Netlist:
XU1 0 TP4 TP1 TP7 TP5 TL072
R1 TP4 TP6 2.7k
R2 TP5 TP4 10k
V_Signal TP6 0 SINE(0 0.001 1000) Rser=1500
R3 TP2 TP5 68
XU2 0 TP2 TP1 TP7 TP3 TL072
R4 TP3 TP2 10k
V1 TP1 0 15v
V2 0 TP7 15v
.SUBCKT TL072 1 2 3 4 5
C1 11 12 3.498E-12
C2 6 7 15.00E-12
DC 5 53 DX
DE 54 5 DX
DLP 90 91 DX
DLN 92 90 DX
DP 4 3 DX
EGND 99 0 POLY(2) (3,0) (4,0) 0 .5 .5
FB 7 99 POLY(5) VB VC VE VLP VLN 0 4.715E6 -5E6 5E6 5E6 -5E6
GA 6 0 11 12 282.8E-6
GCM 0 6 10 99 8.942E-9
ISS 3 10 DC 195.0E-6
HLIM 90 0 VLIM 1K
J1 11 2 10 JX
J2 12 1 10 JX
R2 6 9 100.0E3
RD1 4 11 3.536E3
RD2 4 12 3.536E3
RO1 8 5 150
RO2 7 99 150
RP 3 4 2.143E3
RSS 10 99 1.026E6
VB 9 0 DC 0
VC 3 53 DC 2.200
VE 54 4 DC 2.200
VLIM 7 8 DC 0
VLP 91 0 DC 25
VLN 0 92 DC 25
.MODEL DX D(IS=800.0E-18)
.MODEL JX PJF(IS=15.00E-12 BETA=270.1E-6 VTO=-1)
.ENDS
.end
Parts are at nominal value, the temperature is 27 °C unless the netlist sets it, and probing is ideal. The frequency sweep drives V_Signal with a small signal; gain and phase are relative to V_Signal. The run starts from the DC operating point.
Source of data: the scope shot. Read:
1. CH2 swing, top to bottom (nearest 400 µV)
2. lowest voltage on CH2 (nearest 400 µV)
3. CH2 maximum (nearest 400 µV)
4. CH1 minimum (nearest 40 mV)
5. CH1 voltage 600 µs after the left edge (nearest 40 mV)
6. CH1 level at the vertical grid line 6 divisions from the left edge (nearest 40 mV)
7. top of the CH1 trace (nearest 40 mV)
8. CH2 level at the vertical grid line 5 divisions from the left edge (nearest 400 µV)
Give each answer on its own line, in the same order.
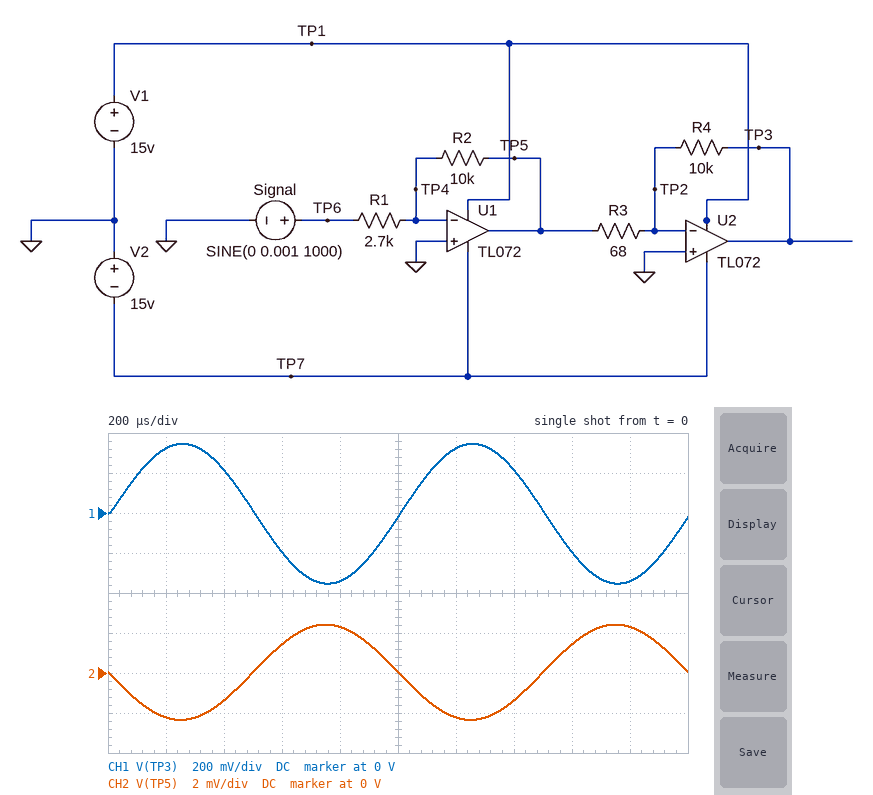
4.8 mV
-2.4 mV
2.4 mV
-360 mV
-200 mV
320 mV
360 mV
0 V
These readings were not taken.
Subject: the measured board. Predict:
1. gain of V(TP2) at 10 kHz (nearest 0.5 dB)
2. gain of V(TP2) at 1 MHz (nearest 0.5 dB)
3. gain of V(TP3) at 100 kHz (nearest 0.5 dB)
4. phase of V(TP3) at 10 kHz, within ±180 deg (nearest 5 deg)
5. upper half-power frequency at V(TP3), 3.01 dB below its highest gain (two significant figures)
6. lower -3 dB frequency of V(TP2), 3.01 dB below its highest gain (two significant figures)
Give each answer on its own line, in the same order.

-0.5 dB
5.0 dB
37.5 dB
-25 deg
22 kHz
21 kHz
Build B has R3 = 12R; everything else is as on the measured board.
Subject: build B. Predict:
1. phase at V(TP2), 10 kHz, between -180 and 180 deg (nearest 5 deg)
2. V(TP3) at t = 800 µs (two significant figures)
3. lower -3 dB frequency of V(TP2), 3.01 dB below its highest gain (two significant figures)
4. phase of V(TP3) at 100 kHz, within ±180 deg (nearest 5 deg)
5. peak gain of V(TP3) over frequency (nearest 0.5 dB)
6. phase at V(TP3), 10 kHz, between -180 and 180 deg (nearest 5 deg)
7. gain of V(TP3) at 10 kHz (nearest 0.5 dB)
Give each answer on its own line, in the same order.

-160 deg
-1.9 V
3.9 kHz
-95 deg
66.0 dB
-70 deg
57.0 dB
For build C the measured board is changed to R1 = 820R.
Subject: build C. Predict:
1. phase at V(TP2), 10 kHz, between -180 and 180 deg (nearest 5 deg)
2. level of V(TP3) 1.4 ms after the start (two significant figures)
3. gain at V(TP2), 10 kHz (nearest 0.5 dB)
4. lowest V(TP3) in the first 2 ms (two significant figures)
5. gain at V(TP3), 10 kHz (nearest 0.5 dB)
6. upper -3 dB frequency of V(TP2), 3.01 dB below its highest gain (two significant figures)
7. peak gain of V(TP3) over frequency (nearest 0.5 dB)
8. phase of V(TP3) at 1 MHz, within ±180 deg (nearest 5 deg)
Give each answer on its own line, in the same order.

-115 deg
390 mV
4.5 dB
-640 mV
55.0 dB
800 kHz
56.0 dB
-160 deg
